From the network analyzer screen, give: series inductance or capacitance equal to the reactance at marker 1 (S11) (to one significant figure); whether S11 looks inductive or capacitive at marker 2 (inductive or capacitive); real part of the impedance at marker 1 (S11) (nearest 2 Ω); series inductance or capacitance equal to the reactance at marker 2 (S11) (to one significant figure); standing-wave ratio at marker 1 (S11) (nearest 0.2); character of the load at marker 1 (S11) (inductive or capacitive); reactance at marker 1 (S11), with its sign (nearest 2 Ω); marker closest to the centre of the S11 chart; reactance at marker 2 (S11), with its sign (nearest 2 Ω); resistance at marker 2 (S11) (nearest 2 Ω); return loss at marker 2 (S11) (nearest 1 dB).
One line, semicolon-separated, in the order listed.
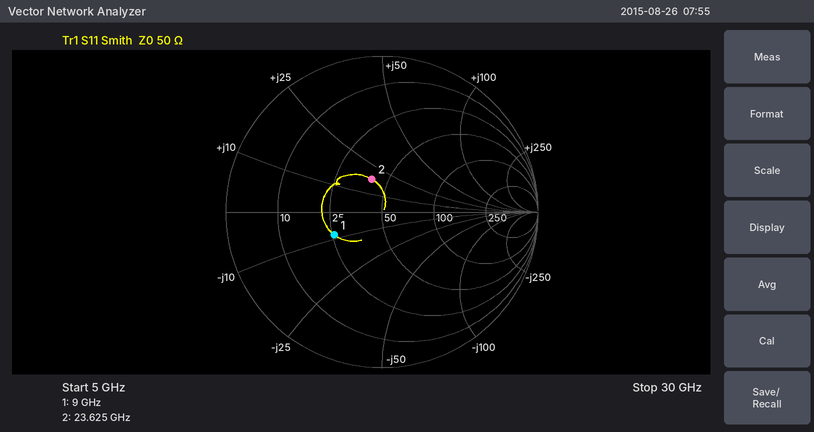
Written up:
2 pF; inductive; 26 Ω; 100 pH; 2.0; capacitive; -8 Ω; marker 2; +18 Ω; 40 Ω; 13 dB
